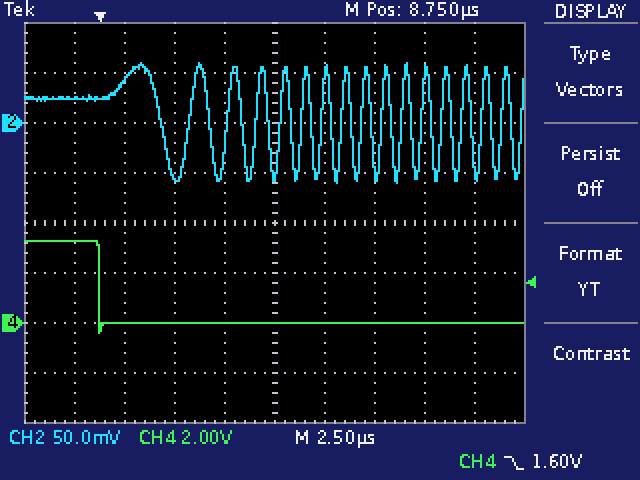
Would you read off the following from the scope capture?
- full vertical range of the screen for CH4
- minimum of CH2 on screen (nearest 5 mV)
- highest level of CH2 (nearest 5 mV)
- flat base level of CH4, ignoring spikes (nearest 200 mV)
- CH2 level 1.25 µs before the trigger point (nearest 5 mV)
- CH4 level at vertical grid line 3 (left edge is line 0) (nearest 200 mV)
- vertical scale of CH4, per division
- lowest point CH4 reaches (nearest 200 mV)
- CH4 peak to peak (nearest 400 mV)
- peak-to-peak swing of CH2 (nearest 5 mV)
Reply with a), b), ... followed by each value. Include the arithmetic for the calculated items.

a) 16 V
b) -60 mV
c) 60 mV
d) 0.0 V
e) 25 mV
f) 0.0 V
g) 2 V
h) -400 mV
i) 3.6 V
j) 60 mV − (-60 mV) = 120 mV
